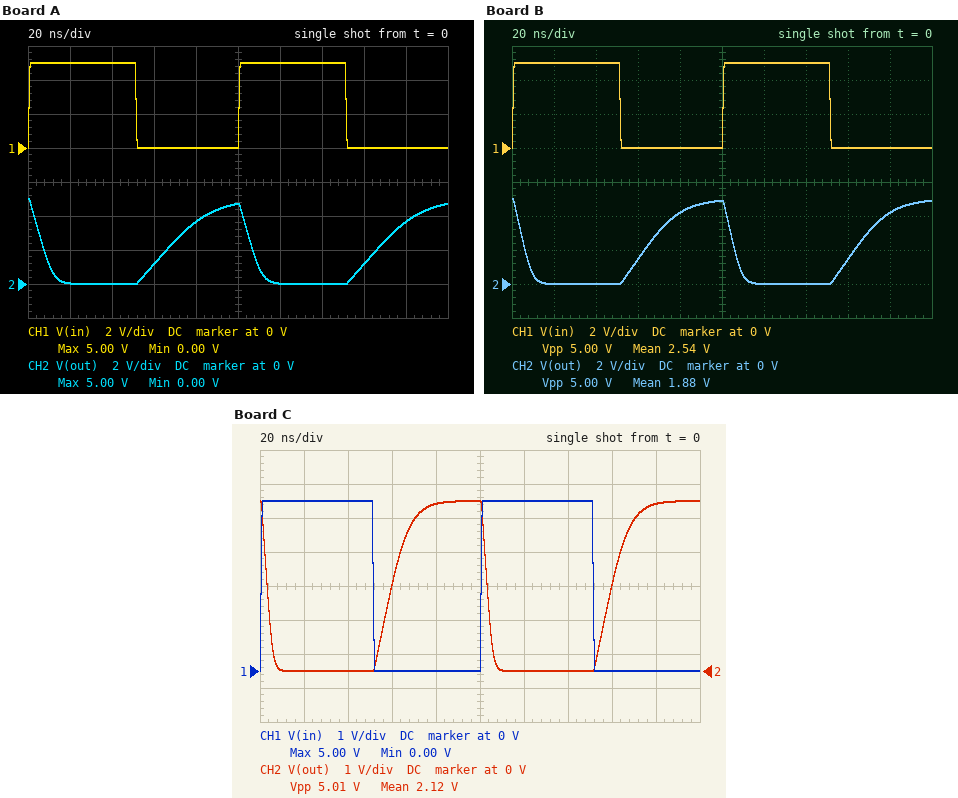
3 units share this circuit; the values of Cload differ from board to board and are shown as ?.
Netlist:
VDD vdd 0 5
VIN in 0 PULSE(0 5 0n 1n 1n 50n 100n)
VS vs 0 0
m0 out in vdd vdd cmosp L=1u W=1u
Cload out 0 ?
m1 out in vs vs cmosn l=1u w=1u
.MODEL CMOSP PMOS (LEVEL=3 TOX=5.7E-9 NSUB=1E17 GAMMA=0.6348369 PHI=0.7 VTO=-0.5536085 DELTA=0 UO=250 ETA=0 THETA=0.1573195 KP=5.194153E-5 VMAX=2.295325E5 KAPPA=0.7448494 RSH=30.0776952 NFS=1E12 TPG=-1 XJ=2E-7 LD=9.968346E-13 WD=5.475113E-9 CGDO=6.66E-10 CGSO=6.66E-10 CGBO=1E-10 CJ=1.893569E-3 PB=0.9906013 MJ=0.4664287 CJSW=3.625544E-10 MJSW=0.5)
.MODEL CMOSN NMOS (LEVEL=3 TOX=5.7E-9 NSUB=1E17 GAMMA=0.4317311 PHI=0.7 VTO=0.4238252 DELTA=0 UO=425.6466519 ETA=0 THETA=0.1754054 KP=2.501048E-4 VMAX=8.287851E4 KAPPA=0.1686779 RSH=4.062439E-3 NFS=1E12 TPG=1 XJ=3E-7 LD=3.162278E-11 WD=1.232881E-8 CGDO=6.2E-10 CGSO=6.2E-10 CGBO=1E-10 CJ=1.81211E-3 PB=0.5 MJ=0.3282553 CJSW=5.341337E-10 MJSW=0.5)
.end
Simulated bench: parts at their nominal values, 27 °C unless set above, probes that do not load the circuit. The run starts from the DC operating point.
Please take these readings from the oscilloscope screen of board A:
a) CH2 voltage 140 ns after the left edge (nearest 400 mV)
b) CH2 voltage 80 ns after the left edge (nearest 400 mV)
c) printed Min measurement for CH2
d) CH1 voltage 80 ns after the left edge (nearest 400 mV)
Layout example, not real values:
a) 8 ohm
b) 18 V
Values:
a) 0 V
b) 3.6 V
c) 0.00 V
d) 0 V
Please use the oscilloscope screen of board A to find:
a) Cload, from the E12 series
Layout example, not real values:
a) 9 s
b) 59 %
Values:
a) 1.5 pF
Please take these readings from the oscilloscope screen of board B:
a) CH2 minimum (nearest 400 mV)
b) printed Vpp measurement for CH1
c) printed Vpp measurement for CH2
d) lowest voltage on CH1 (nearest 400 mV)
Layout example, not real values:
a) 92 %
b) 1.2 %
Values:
a) 0 V
b) 5.00 V
c) 5.00 V
d) 0 V
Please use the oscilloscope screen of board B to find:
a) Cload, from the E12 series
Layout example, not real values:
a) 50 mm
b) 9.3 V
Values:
a) 1.2 pF
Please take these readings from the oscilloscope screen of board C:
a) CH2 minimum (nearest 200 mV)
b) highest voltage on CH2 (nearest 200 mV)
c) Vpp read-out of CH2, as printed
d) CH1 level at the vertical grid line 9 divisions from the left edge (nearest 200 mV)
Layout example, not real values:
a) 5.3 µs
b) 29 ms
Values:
a) 0 V
b) 5.0 V
c) 5.01 V
d) 0 V
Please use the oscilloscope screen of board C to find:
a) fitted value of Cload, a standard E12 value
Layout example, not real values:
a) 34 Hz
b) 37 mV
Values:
a) 680 fF
